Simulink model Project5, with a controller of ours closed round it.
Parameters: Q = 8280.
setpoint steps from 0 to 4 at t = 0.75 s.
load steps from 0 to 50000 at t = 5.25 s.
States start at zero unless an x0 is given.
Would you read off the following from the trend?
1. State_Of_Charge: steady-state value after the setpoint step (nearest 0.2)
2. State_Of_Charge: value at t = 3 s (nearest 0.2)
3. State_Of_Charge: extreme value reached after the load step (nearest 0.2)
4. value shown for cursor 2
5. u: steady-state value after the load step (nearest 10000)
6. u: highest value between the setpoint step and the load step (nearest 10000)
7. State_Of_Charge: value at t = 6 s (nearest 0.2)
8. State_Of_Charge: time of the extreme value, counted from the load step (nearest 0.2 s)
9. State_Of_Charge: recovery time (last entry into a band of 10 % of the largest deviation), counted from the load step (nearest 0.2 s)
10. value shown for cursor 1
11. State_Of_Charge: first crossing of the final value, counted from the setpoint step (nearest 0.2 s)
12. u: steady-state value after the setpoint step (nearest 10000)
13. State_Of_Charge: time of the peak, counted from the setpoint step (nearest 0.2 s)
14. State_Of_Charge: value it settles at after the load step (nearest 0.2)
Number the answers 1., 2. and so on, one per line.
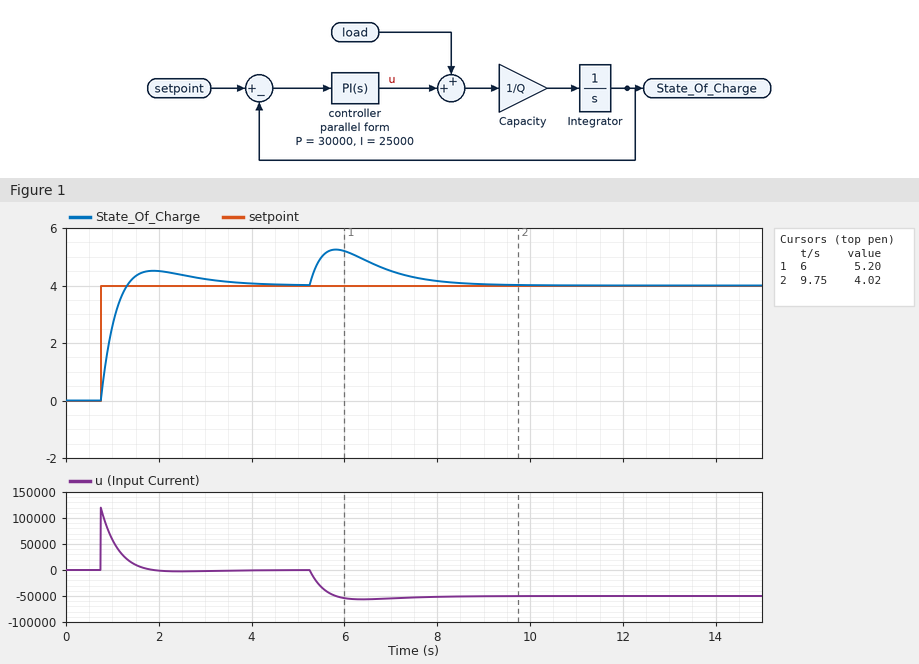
1. 4.0
2. 4.2
3. 5.2
4. 4.02
5. -50000
6. 120000
7. 5.2
8. 0.6 s
9. 3.0 s
10. 5.20
11. 0.6 s
12. 0
13. 1.2 s
14. 4.0
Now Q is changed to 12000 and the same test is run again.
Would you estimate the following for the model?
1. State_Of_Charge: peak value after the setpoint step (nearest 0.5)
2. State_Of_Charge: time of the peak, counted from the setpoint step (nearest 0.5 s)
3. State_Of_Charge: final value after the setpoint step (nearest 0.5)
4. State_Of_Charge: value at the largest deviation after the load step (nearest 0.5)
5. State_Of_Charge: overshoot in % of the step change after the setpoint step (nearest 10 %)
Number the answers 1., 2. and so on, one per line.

1. 4.5
2. 1.5 s
3. 4.0
4. 5.0
5. 20 %
